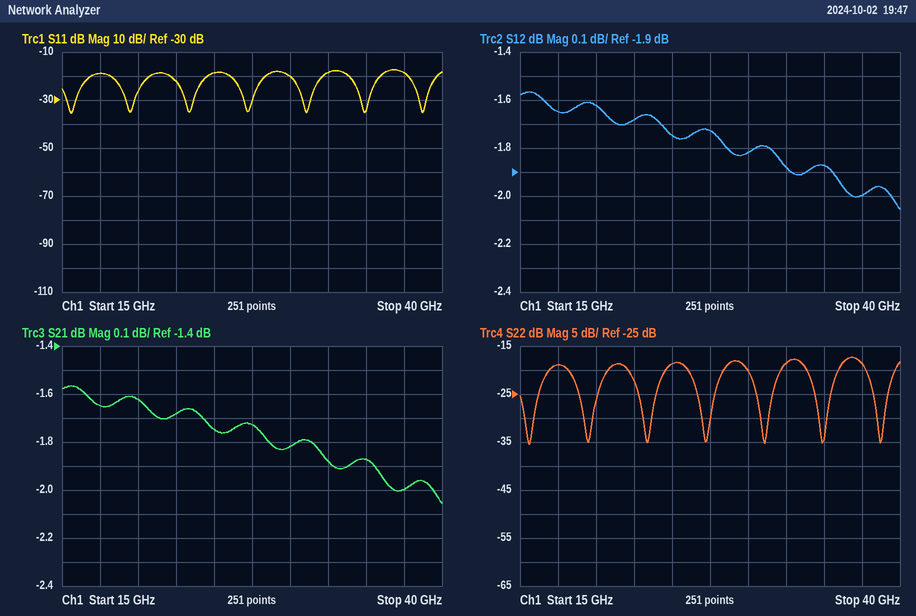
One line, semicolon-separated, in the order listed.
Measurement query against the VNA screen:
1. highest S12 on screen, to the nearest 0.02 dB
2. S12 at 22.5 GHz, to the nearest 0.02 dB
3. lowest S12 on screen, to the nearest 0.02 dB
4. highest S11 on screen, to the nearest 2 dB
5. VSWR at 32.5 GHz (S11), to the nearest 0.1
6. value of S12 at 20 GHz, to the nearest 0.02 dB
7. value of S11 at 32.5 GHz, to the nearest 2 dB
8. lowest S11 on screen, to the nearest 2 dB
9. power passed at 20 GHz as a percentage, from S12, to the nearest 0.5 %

-1.56 dB; -1.68 dB; -2.06 dB; -18 dB; 1.3; -1.62 dB; -18 dB; -36 dB; 69.0 %
